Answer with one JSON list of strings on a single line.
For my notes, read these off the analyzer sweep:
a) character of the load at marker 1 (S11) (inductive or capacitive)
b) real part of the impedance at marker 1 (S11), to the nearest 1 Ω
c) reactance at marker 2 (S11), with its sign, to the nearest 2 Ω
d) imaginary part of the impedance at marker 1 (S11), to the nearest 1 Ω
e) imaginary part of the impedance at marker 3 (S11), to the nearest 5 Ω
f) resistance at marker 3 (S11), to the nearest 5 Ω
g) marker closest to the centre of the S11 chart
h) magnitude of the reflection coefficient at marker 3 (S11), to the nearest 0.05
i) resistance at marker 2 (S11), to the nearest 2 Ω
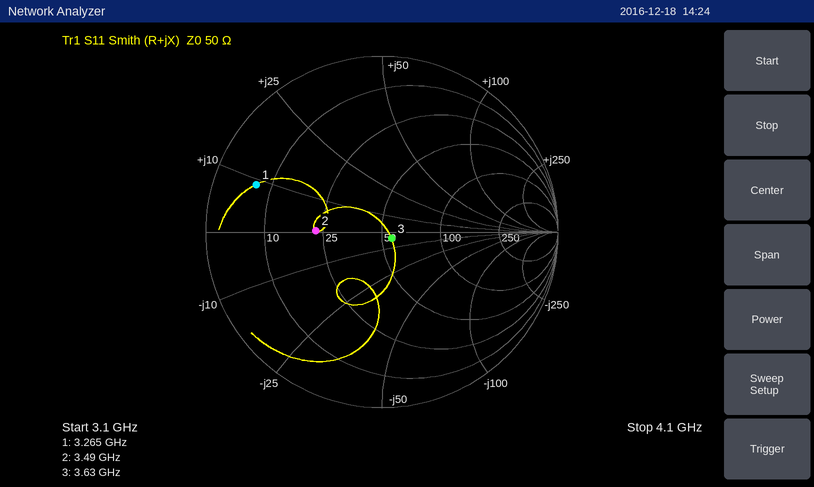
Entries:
["inductive", "7 Ω", "0 Ω", "+9 Ω", "-5 Ω", "55 Ω", "marker 3", "0.05", "22 Ω"]
